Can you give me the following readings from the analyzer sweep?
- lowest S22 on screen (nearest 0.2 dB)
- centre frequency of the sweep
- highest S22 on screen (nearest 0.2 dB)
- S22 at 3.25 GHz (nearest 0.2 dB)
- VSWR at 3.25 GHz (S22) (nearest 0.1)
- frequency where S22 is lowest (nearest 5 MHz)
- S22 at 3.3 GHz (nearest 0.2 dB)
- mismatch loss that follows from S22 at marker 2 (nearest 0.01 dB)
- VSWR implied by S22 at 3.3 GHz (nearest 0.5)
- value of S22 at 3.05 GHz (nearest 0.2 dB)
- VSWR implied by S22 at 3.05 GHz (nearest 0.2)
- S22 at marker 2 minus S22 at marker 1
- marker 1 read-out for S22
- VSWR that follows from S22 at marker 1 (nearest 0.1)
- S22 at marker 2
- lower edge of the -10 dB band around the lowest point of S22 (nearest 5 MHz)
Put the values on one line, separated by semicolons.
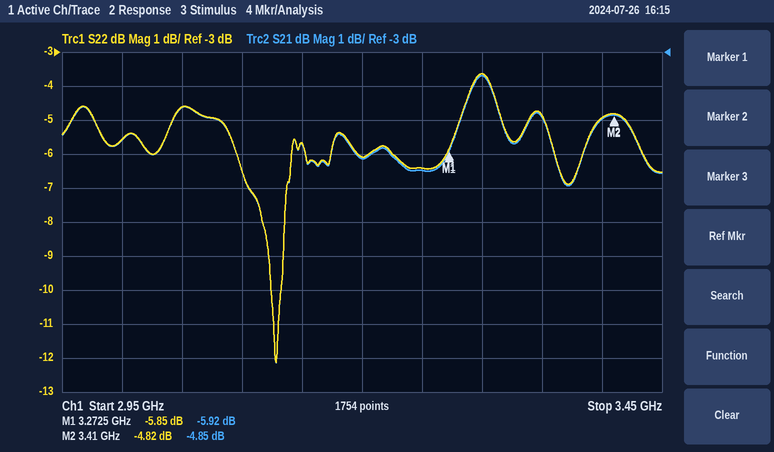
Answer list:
-12.2 dB; 3.2 GHz; -3.6 dB; -6.4 dB; 2.8; 3.130 GHz; -3.6 dB; 1.74 dB; 5.0; -4.6 dB; 3.8; 1.03 dB; -5.85 dB; 3.1; -4.82 dB; 3.125 GHz
